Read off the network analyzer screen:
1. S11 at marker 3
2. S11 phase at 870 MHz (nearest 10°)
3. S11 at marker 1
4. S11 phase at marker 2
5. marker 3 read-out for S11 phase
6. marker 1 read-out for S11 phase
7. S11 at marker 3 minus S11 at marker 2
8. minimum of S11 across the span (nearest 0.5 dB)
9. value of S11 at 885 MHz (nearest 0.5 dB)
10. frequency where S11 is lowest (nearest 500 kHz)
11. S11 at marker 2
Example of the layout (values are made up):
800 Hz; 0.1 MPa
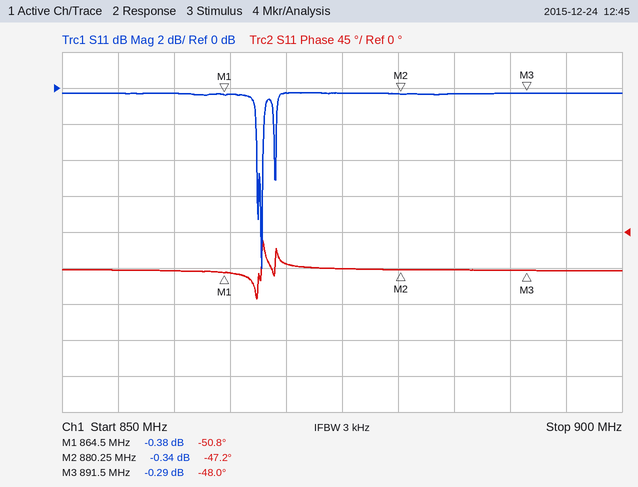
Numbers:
-0.29 dB; -40°; -0.38 dB; -47.2°; -48.0°; -50.8°; 0.05 dB; -10.0 dB; -0.5 dB; 868.0 MHz; -0.34 dB
